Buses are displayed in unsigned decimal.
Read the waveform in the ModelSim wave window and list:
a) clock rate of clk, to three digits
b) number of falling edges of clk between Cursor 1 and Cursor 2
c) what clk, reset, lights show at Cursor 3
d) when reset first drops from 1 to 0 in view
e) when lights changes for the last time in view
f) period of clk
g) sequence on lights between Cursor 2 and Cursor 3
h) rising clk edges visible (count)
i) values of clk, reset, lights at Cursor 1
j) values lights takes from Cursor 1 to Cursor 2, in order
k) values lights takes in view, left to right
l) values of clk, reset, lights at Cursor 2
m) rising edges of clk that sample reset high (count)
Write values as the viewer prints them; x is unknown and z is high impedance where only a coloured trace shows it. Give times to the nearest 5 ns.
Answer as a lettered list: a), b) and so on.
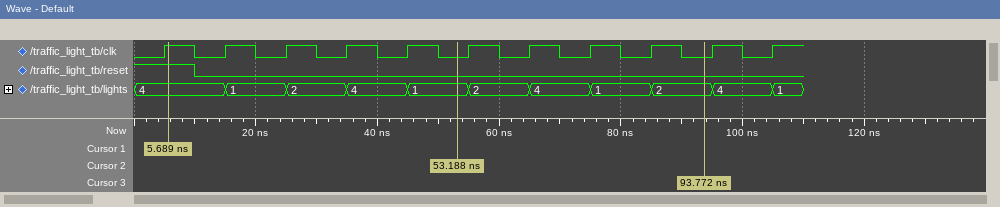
a) 100 MHz
b) 5
c) clk=0, reset=0, lights=2
d) 10 ns
e) 105 ns
f) 10 ns
g) 1, 2, 4, 1, 2
h) 11
i) clk=1, reset=1, lights=4
j) 4, 1, 2, 4, 1
k) 4, 1, 2, 4, 1, 2, 4, 1, 2, 4, 1
l) clk=0, reset=0, lights=1
m) 1
